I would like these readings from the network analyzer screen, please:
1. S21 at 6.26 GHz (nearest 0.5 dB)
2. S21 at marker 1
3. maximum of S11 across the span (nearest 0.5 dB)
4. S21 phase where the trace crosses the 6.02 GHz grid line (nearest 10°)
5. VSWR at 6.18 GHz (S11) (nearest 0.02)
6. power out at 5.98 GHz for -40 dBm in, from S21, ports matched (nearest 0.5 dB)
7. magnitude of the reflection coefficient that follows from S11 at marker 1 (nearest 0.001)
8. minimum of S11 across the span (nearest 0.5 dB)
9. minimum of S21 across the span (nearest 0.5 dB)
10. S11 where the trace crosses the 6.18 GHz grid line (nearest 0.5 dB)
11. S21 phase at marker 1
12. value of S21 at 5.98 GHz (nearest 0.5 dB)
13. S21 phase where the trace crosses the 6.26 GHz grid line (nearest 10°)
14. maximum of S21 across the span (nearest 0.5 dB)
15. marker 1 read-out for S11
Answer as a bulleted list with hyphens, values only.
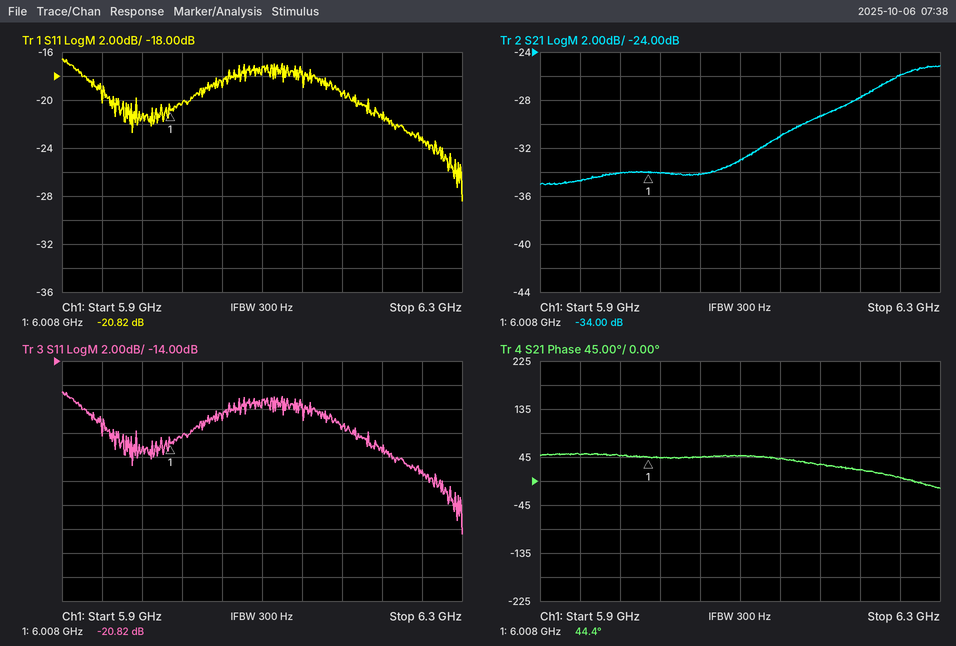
- -26.0 dB
- -34.00 dB
- -16.5 dB
- 40°
- 1.24
- -74.0 dBm
- 0.091
- -28.5 dB
- -35.0 dB
- -19.5 dB
- 44.4°
- -34.0 dB
- 10°
- -25.0 dB
- -20.82 dB
